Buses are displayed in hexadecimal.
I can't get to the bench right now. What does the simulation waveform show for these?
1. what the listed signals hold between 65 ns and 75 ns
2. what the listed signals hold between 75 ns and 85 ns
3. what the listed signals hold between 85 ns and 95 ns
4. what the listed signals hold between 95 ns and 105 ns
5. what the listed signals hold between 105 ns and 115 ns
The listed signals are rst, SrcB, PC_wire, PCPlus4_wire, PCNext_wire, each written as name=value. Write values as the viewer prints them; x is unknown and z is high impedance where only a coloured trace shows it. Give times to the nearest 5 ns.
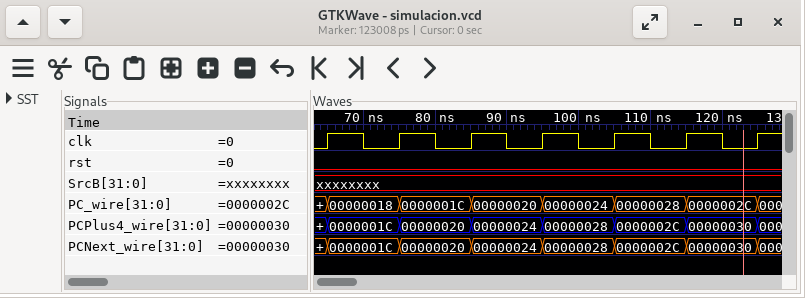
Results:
rst=0, SrcB=xxxxxxxx, PC_wire=00000018, PCPlus4_wire=0000001C, PCNext_wire=0000001C
rst=0, SrcB=xxxxxxxx, PC_wire=0000001C, PCPlus4_wire=00000020, PCNext_wire=00000020
rst=0, SrcB=xxxxxxxx, PC_wire=00000020, PCPlus4_wire=00000024, PCNext_wire=00000024
rst=0, SrcB=xxxxxxxx, PC_wire=00000024, PCPlus4_wire=00000028, PCNext_wire=00000028
rst=0, SrcB=xxxxxxxx, PC_wire=00000028, PCPlus4_wire=0000002C, PCNext_wire=0000002C
